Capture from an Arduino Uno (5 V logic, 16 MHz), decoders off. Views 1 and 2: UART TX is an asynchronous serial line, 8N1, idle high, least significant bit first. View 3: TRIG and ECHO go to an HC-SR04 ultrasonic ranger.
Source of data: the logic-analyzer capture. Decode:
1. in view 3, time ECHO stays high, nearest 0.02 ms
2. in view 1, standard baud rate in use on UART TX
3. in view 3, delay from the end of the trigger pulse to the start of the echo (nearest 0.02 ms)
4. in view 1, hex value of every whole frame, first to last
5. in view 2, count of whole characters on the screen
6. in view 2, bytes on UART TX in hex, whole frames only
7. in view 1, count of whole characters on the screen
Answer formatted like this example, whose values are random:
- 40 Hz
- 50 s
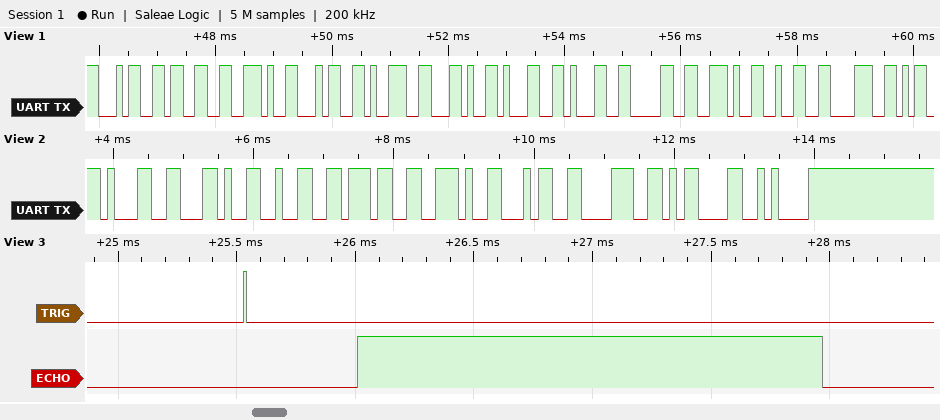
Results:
- 1.96 ms
- 9600 baud
- 0.46 ms
- 34 33 2E 34 39 2C 31 31 30 2E 32 38
- 9
- 31 2C 32 37 2E 34 38 0D 0A
- 12
